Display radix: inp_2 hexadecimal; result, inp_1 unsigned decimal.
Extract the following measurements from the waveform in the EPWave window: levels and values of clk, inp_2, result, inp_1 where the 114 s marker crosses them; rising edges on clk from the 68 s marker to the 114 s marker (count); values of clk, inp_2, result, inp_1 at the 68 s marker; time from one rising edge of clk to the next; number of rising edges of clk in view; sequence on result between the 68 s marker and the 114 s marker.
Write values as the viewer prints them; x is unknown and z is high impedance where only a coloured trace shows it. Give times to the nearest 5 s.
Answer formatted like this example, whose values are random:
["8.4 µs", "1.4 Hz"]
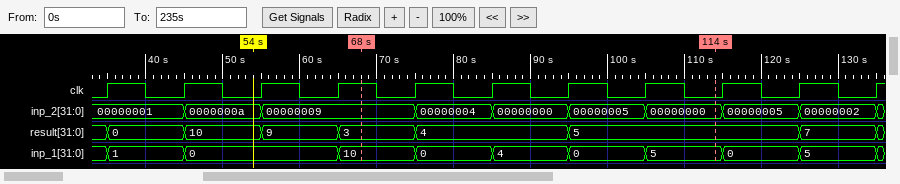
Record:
["clk=0, inp_2=00000000, result=5, inp_1=5", "4", "clk=1, inp_2=00000009, result=3, inp_1=10", "10 s", "11", "3, 4, 5"]
